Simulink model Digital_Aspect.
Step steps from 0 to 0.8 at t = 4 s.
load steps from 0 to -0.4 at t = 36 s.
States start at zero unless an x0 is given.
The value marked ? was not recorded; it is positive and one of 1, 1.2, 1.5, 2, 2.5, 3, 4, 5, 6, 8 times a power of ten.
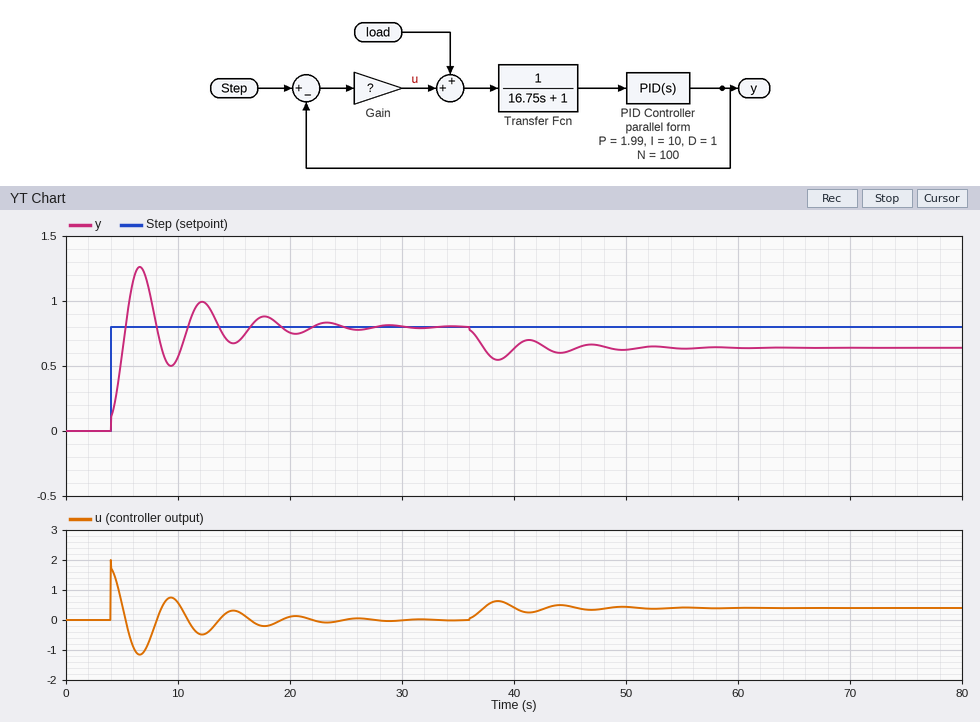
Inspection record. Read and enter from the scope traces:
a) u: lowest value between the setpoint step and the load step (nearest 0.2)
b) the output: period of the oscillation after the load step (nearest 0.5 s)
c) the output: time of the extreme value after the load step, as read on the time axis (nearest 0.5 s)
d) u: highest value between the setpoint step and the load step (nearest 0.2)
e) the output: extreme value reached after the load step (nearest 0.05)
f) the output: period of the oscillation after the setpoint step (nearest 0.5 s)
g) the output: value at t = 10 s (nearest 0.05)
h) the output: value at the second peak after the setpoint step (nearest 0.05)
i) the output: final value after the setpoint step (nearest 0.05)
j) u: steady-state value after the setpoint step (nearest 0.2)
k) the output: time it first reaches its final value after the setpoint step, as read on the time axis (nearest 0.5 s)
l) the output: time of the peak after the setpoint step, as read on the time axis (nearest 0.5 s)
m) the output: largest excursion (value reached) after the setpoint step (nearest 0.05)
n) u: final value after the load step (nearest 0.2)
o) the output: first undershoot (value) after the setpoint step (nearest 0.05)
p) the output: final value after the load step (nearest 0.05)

-1.2
5.5 s
38.5 s
2.0
0.55
5.5 s
0.55
1.00
0.80
0.0
5.5 s
6.5 s
1.25
0.4
0.50
0.65
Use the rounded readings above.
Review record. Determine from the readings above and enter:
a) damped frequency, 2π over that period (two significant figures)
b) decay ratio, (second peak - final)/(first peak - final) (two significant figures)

1.1 rad/s
0.44
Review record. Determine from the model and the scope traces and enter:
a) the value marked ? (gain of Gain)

2.5
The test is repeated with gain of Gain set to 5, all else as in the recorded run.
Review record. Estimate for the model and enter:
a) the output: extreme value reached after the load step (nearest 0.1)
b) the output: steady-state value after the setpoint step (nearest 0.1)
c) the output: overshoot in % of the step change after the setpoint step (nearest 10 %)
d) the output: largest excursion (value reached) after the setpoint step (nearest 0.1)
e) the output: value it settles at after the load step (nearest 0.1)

0.7
0.8
50 %
1.2
0.7
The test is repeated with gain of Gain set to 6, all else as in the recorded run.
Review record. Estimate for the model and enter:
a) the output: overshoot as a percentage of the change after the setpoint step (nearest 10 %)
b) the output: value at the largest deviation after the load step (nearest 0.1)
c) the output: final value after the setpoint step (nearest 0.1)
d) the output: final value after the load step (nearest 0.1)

40 %
0.7
0.8
0.7
